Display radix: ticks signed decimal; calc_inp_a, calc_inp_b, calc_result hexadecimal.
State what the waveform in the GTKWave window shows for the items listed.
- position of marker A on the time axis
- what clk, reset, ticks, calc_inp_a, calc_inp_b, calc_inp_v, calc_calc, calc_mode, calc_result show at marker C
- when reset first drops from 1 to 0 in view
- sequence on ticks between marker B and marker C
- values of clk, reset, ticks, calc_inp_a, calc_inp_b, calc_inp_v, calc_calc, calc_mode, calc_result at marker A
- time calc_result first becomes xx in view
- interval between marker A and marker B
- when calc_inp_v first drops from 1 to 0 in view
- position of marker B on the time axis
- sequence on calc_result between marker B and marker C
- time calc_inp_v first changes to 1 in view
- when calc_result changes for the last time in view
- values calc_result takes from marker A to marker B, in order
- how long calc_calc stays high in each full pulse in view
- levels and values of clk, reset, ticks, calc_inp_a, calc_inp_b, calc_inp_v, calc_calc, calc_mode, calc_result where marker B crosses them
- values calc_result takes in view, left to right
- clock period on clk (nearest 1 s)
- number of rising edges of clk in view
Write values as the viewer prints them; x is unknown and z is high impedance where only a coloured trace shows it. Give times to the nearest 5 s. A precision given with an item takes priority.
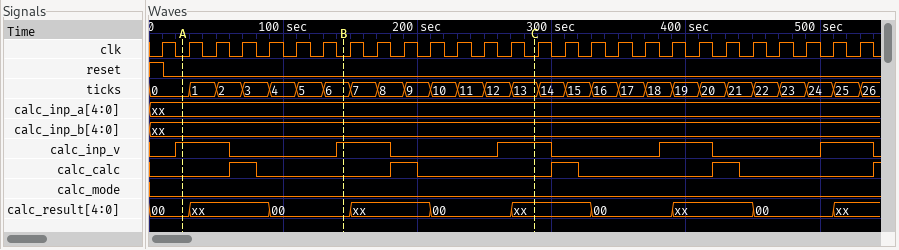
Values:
25 s
clk=0, reset=0, ticks=13, calc_inp_a=xx, calc_inp_b=xx, calc_inp_v=1, calc_calc=0, calc_mode=0, calc_result=xx
10 s
6, 7, 8, 9, 10, 11, 12, 13
clk=0, reset=0, ticks=0, calc_inp_a=xx, calc_inp_b=xx, calc_inp_v=1, calc_calc=0, calc_mode=0, calc_result=00
30 s
120 s
60 s
145 s
00, xx, 00, xx
20 s
510 s
00, xx, 00
20 s, 20 s, 20 s, 20 s
clk=0, reset=0, ticks=6, calc_inp_a=xx, calc_inp_b=xx, calc_inp_v=1, calc_calc=0, calc_mode=0, calc_result=00
00, xx, 00, xx, 00, xx, 00, xx, 00, xx
20 s
27
